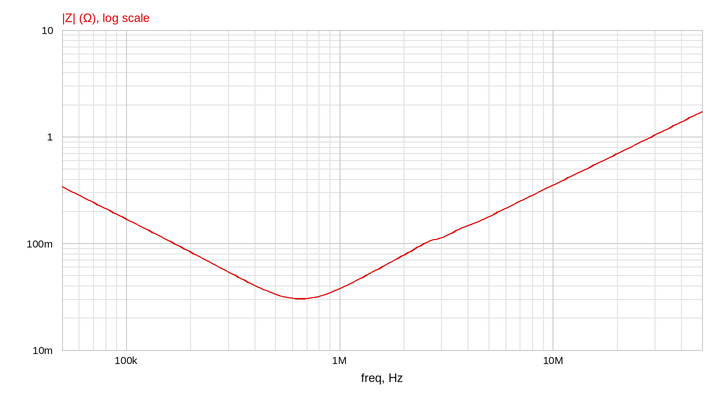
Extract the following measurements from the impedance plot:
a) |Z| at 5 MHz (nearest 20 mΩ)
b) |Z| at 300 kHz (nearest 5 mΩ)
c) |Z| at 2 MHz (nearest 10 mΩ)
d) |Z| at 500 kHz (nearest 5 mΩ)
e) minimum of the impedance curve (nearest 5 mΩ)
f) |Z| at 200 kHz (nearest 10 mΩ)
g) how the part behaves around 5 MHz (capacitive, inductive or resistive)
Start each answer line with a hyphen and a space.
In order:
- 180 mΩ
- 55 mΩ
- 80 mΩ
- 35 mΩ
- 30 mΩ
- 80 mΩ
- inductive
